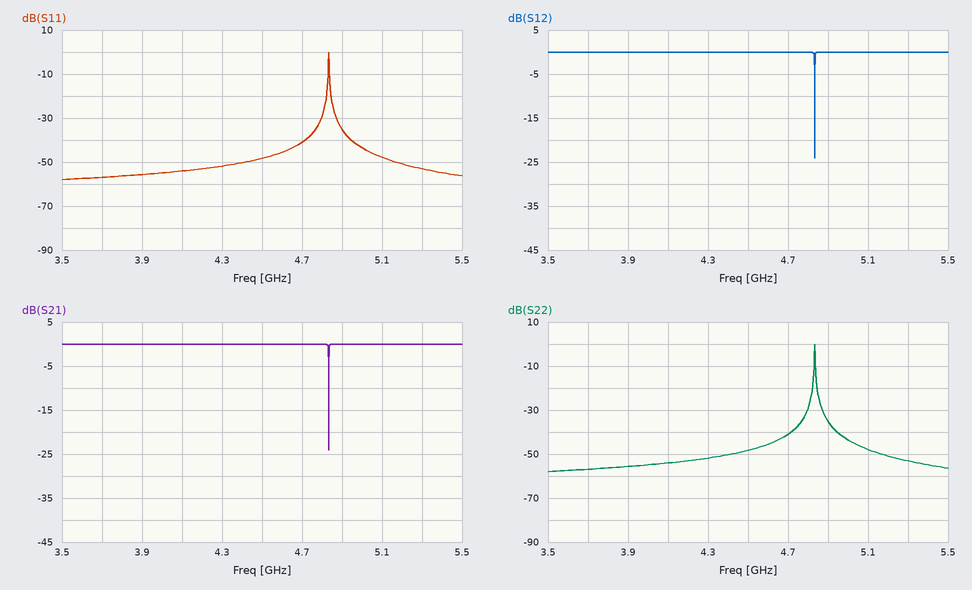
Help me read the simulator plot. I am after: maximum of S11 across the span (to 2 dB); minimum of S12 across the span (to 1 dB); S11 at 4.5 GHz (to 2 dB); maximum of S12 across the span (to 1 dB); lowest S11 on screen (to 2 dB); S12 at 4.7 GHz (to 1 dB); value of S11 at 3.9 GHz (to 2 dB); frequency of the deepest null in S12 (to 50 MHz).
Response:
0 dB
-24 dB
-48 dB
0 dB
-58 dB
0 dB
-56 dB
4.85 GHz
